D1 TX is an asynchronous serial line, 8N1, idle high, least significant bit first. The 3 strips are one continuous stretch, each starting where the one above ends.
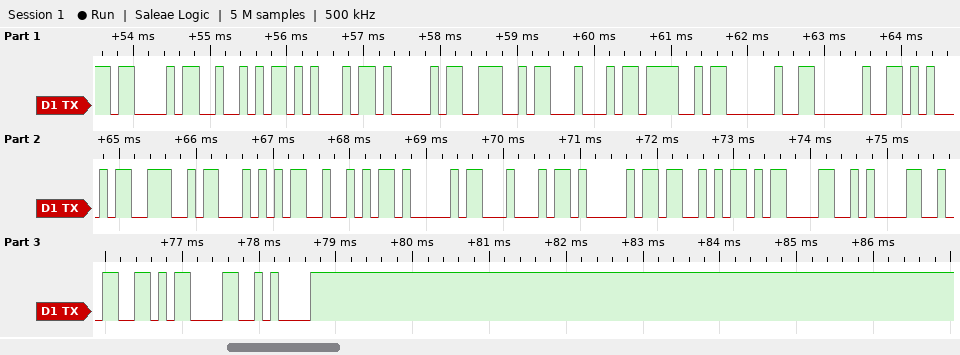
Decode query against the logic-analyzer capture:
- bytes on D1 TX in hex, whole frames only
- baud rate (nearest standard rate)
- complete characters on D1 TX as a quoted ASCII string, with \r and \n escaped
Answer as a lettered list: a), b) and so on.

a) 43 52 45 41 4E 44 4F 20 20 45 4E 54 52 41 44 41 53 0D 0A 32 0D 0A
b) 9600 baud
c) "CREANDO  ENTRADAS\r\n2\r\n"
